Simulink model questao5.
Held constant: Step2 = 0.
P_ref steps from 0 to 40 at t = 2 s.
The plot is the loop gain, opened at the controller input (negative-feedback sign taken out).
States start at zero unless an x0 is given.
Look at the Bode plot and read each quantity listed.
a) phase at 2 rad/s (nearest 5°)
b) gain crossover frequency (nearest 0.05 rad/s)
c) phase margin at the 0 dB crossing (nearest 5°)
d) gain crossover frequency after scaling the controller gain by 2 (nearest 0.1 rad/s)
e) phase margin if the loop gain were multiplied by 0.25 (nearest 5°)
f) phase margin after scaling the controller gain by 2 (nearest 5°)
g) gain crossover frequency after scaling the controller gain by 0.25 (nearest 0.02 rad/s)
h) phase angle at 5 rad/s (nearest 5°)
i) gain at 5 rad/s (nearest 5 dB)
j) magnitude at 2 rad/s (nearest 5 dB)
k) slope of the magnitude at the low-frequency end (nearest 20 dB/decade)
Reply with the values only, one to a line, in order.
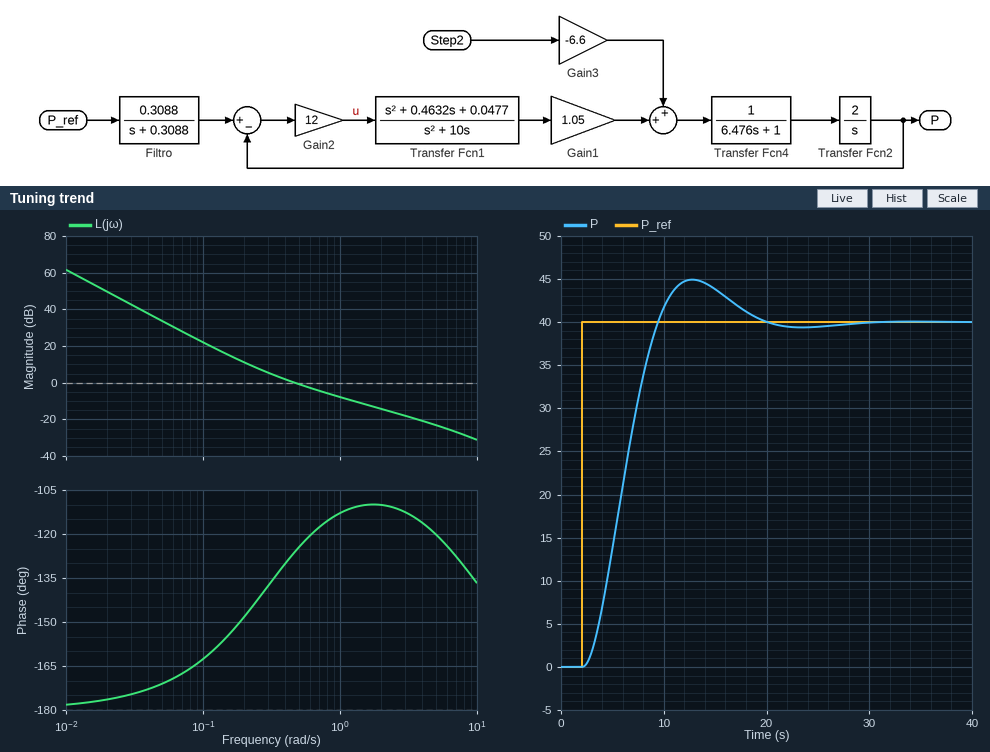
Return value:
-110°
0.45 rad/s
55°
0.8 rad/s
30°
65°
0.18 rad/s
-120°
-25 dB
-15 dB
-40 dB/decade
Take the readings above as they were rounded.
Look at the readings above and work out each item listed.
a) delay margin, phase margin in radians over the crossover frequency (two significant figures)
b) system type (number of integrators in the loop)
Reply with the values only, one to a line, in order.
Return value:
2.1 s
2
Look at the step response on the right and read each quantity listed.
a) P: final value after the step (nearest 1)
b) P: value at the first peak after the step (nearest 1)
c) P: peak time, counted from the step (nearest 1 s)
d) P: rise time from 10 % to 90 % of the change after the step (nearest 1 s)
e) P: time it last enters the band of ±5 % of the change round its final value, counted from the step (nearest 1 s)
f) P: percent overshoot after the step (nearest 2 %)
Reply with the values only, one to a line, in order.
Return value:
40
45
11 s
5 s
15 s
12 %
